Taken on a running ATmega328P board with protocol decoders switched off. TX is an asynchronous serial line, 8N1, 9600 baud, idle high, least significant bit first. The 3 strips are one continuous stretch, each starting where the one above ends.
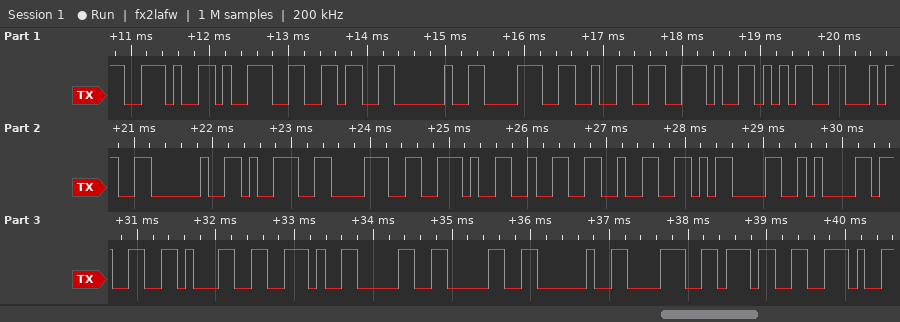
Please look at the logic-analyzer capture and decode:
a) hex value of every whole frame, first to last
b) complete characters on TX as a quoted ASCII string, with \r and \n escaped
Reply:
2E 39 36 20 38 32 2E 35 34 20 39 38 2E 32 32 0D 0A 33 31 2E 30 30 20 38 37 2E
".96 82.54 98.22\r\n31.00 87."
